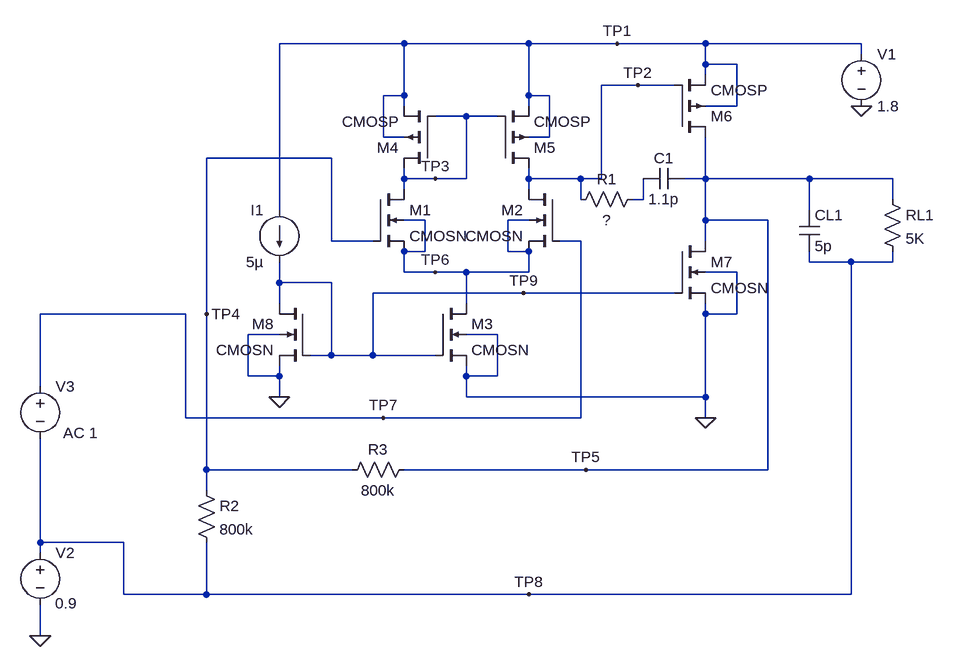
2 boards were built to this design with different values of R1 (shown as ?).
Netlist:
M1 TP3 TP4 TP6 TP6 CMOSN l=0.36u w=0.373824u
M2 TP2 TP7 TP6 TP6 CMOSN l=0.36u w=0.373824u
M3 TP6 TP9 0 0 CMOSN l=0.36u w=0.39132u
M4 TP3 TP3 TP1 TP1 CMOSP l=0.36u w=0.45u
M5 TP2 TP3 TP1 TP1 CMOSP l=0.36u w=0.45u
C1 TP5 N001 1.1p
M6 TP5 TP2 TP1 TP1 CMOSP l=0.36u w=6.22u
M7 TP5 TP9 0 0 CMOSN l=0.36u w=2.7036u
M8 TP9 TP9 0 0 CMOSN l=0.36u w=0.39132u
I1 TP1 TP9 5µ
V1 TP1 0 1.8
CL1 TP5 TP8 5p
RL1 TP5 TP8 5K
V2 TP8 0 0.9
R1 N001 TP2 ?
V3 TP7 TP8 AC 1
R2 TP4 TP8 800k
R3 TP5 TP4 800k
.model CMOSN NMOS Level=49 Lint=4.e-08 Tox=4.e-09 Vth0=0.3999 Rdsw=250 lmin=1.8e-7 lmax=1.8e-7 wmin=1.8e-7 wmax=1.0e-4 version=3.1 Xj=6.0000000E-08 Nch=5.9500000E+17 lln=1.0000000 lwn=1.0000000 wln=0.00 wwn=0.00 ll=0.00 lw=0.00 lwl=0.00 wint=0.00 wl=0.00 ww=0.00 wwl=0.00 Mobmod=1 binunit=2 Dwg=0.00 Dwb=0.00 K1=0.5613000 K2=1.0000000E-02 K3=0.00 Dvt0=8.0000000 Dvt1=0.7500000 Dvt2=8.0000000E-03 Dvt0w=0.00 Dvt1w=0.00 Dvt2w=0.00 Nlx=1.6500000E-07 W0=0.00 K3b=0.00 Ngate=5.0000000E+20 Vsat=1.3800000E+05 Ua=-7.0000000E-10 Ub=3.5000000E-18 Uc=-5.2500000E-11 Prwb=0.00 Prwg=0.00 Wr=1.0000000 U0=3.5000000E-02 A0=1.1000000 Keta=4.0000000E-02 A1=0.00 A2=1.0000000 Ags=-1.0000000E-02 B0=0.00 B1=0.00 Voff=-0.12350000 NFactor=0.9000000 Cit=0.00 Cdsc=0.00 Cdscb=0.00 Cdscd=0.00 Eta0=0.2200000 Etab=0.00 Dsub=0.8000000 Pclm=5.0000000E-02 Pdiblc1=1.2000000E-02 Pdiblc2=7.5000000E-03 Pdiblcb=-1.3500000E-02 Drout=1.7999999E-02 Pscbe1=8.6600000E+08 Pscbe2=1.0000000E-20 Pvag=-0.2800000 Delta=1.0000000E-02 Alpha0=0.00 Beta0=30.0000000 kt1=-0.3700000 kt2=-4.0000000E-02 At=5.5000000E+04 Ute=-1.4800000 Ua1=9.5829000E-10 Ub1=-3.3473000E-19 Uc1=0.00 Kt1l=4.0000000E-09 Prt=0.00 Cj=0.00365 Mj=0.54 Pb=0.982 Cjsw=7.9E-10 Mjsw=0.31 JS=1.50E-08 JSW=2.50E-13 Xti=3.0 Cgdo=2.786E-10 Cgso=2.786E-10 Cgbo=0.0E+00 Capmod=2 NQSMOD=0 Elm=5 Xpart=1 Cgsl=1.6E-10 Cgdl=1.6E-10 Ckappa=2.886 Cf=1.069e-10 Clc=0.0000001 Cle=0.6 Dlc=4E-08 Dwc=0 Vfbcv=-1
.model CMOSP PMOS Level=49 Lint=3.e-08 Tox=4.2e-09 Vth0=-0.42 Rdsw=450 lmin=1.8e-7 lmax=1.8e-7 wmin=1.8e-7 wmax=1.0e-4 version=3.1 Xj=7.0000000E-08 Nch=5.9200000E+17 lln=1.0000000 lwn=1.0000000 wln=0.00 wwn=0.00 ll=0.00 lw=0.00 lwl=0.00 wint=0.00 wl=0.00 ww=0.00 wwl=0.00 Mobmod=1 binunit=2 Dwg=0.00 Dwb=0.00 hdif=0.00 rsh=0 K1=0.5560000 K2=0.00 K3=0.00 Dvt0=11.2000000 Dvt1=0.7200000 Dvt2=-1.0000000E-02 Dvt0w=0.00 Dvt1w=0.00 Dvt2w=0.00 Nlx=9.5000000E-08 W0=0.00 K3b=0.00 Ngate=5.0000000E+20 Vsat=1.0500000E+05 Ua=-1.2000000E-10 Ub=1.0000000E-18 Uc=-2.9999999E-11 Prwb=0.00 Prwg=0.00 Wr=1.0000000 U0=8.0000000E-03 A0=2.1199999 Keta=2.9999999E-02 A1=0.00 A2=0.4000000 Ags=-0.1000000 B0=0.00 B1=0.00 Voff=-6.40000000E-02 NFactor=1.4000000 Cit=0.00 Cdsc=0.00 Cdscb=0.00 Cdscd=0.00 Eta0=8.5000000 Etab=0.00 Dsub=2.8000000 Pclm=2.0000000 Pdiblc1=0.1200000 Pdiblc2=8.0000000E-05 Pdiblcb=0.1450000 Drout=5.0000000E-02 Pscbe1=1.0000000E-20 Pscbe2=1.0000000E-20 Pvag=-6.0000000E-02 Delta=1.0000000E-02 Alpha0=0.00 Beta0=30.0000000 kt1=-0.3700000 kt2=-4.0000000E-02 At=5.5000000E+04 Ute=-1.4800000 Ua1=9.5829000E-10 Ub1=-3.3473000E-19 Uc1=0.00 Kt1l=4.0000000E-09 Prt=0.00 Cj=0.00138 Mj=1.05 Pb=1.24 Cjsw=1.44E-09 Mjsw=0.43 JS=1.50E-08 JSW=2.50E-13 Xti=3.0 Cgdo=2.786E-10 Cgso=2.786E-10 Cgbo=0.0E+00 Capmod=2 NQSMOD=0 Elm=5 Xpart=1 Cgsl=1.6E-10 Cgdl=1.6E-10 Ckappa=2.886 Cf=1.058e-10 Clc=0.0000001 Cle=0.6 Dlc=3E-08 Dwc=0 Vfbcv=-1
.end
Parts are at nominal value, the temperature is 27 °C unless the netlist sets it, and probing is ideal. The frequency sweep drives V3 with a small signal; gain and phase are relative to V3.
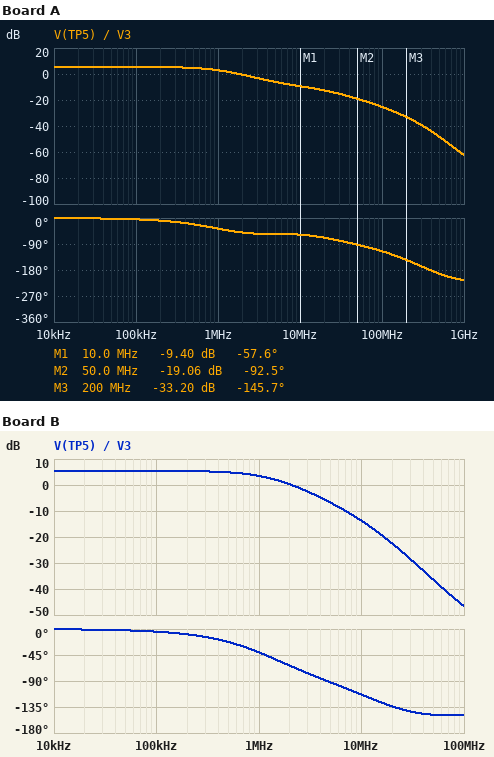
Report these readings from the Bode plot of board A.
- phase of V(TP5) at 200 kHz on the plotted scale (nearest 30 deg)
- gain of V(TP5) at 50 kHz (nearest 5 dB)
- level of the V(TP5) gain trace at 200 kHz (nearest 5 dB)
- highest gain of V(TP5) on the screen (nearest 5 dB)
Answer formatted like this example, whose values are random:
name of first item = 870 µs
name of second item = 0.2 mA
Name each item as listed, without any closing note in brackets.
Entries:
phase of V(TP5) at 200 kHz on the plotted scale = 0 deg
gain of V(TP5) at 50 kHz = 5 dB
level of the V(TP5) gain trace at 200 kHz = 5 dB
highest gain of V(TP5) on the screen = 5 dB
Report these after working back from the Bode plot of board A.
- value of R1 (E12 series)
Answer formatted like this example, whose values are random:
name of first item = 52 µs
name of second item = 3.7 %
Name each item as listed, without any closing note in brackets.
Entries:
value of R1 = 27 kΩ
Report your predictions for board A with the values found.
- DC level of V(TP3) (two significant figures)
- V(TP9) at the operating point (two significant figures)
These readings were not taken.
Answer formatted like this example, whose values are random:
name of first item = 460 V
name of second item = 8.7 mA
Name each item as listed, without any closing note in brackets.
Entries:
DC level of V(TP3) = 1.1 V
V(TP9) at the operating point = 680 mV
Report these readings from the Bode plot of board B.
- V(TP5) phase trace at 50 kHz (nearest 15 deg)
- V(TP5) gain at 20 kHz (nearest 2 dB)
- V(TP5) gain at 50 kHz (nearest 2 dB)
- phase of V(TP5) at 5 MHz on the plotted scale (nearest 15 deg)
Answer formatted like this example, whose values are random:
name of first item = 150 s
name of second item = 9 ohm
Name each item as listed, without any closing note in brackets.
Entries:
V(TP5) phase trace at 50 kHz = 0 deg
V(TP5) gain at 20 kHz = 6 dB
V(TP5) gain at 50 kHz = 6 dB
phase of V(TP5) at 5 MHz on the plotted scale = -90 deg
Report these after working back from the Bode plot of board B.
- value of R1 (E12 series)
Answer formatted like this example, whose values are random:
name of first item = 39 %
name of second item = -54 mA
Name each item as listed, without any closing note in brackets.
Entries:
value of R1 = 4.7 kΩ
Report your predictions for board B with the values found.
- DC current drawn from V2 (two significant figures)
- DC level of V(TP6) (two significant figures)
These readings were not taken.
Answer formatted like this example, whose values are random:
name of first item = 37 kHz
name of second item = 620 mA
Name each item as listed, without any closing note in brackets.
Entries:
DC current drawn from V2 = 160 nA
DC level of V(TP6) = 290 mV
